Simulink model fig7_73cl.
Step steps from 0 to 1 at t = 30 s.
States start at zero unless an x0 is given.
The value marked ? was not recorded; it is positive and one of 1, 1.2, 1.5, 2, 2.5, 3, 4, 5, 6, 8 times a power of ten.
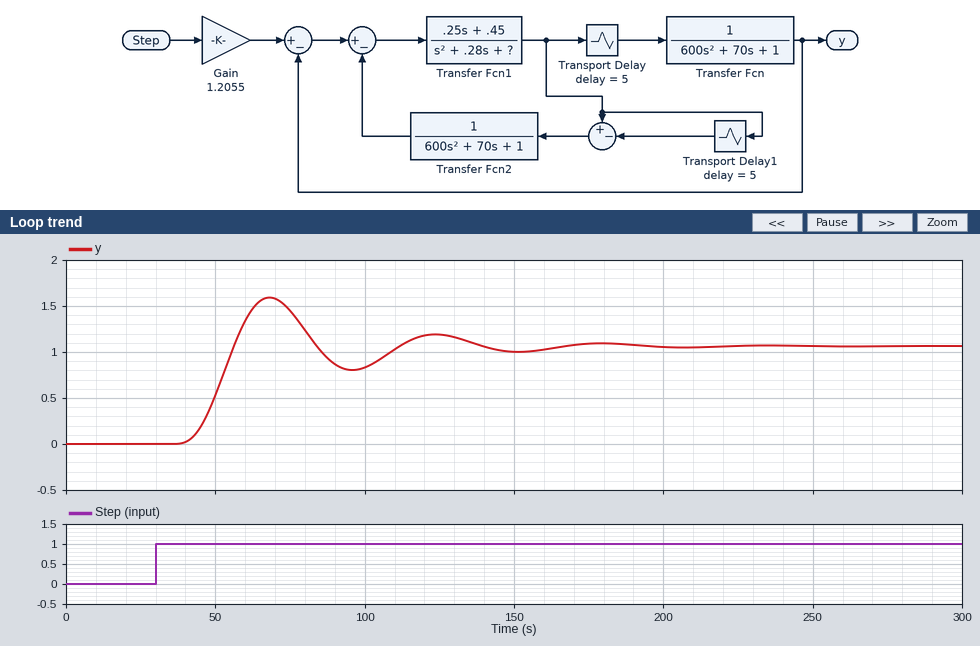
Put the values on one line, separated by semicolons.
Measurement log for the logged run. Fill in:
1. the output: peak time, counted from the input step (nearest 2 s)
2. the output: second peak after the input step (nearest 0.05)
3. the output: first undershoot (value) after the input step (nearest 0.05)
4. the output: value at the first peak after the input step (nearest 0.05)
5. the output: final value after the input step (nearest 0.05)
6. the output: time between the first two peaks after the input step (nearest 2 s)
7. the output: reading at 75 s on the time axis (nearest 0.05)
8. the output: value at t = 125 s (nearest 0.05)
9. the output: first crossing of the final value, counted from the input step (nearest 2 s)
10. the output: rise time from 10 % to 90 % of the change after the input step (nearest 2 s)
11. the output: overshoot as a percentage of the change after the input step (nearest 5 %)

38 s; 1.20; 0.80; 1.60; 1.05; 56 s; 1.45; 1.20; 26 s; 12 s; 50 %
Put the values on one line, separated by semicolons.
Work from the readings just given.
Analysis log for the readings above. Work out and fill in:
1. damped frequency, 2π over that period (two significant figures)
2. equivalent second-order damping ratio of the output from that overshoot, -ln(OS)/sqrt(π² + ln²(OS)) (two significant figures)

0.11 rad/s; 0.22
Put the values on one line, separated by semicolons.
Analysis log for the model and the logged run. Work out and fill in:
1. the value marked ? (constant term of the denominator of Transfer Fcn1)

0.06
